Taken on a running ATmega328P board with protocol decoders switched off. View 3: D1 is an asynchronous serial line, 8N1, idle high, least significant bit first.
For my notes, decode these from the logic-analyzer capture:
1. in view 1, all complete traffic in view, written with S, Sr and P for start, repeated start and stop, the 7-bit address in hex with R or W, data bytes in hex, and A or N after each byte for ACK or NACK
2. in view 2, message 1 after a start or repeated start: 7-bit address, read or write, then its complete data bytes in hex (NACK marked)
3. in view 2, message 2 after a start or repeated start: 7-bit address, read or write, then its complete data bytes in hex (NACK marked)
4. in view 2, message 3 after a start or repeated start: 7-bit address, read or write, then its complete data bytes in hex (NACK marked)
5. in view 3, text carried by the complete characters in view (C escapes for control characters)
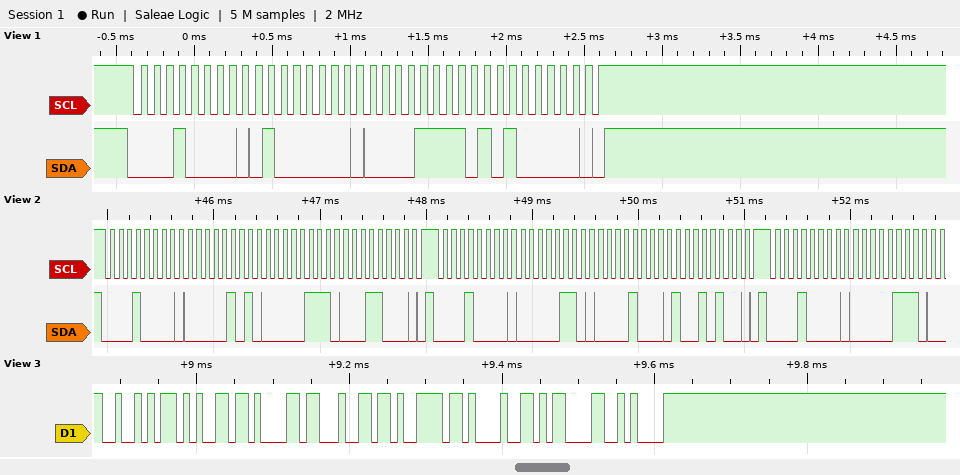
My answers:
S 08W A 40 A 0F A A0 A P
0x08 write: 05 07 18
0x08 write: 06 08 94
0x08 write: 07
"Ready!\r\n"
